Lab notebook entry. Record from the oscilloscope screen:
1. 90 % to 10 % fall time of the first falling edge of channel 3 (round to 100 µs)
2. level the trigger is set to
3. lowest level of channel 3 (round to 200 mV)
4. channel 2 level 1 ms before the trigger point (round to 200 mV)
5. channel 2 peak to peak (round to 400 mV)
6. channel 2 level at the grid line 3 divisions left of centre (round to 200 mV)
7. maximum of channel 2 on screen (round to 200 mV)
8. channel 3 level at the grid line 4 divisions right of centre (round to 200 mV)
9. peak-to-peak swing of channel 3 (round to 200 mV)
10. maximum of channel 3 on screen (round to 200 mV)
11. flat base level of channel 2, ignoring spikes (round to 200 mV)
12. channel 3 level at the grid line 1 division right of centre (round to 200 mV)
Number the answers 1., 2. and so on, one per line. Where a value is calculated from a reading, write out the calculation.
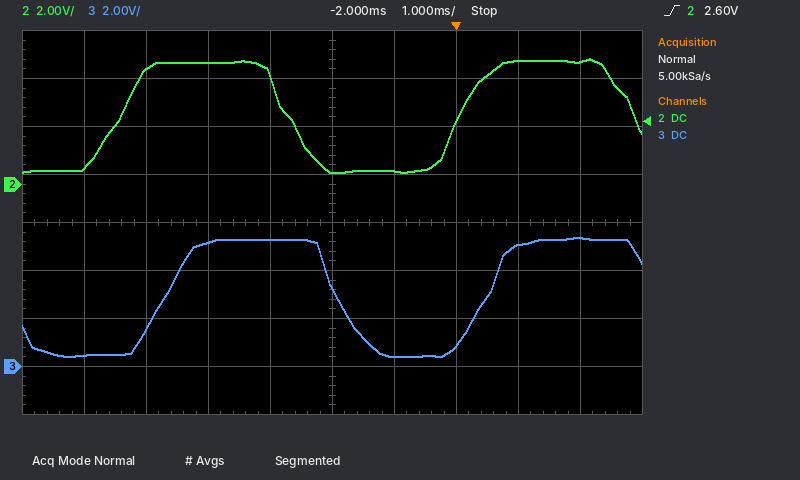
1. 800 µs
2. 2.60 V
3. 400 mV
4. 600 mV
5. 4.8 V
6. 4.8 V
7. 5.2 V
8. 5.4 V
9. 5.4 V − (400 mV) = 5.0 V
10. 5.4 V
11. 600 mV
12. 400 mV
